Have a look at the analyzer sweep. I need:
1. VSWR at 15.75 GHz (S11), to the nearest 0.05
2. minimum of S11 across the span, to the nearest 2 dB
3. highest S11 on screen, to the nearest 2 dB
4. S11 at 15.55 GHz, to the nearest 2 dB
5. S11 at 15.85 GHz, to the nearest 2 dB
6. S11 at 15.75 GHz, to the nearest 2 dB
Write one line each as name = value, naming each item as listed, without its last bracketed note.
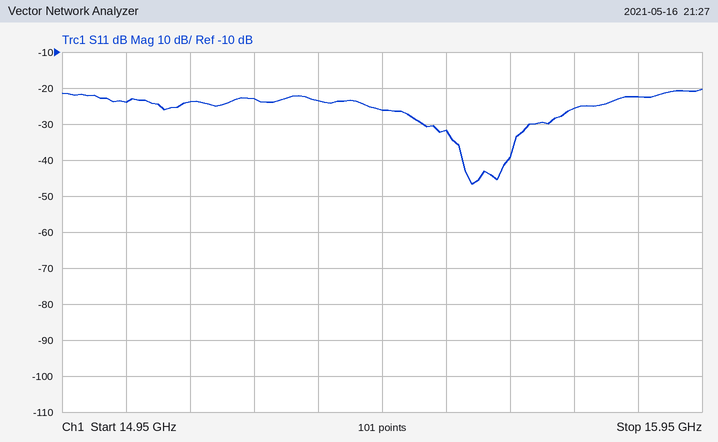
VSWR at 15.75 GHz (S11), to the nearest 0.05 = 1.10
minimum of S11 across the span, to the nearest 2 dB = -46 dB
highest S11 on screen, to the nearest 2 dB = -20 dB
S11 at 15.55 GHz, to the nearest 2 dB = -32 dB
S11 at 15.85 GHz, to the nearest 2 dB = -22 dB
S11 at 15.75 GHz, to the nearest 2 dB = -26 dB
